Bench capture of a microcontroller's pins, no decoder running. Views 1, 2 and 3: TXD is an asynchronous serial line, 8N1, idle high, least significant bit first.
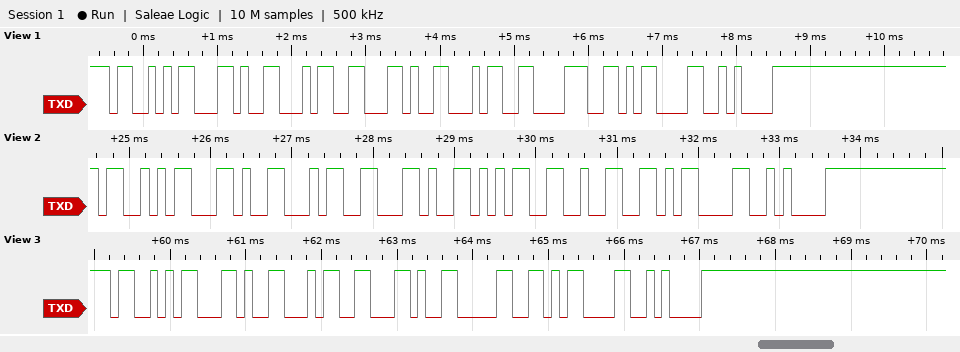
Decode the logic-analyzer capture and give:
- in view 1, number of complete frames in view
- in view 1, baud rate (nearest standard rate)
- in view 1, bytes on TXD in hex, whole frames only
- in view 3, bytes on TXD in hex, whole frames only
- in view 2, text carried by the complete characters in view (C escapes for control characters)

8
9600 baud
0x53 0x2C 0x34 0x2C 0x34 0x38 0x0D 0x0A
53 2C 34 2C 30 0D 0A
"S,4,52\r\n"
